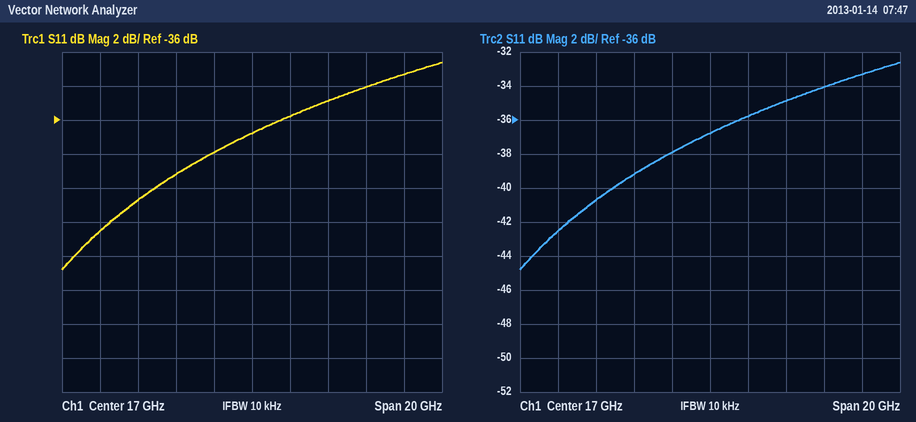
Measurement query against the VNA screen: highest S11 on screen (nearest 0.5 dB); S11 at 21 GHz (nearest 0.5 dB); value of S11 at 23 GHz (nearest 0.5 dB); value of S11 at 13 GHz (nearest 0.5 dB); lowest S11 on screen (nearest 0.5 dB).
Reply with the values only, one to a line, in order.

-32.5 dB
-35.0 dB
-34.0 dB
-39.0 dB
-45.0 dB
